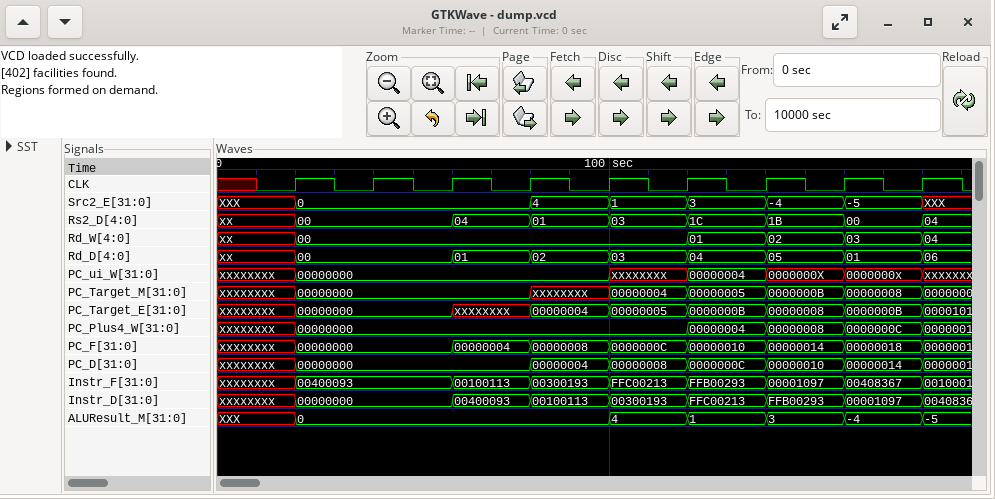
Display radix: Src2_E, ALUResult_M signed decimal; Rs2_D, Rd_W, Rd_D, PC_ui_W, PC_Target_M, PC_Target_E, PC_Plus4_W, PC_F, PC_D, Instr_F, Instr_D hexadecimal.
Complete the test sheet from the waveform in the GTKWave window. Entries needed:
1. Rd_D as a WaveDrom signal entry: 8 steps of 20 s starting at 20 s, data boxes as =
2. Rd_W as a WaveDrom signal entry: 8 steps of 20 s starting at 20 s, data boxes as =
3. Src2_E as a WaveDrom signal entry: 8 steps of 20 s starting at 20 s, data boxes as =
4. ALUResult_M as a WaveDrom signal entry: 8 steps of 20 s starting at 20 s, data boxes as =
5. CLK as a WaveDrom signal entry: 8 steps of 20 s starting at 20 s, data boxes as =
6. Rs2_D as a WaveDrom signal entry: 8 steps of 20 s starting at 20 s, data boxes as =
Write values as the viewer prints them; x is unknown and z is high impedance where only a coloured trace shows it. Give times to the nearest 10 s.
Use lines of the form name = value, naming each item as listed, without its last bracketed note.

Rd_D as a WaveDrom signal entry: 8 steps of 20 s starting at 20 s, data boxes as = = {name: 'Rd_D', wave: '=.======', data: '00 01 02 03 04 05 01'}
Rd_W as a WaveDrom signal entry: 8 steps of 20 s starting at 20 s, data boxes as = = {name: 'Rd_W', wave: '=....===', data: '00 01 02 03'}
Src2_E as a WaveDrom signal entry: 8 steps of 20 s starting at 20 s, data boxes as = = {name: 'Src2_E', wave: '=..=====', data: '0 4 1 3 -4 -5'}
ALUResult_M as a WaveDrom signal entry: 8 steps of 20 s starting at 20 s, data boxes as = = {name: 'ALUResult_M', wave: '=...====', data: '0 4 1 3 -4'}
CLK as a WaveDrom signal entry: 8 steps of 20 s starting at 20 s, data boxes as = = {name: 'CLK', wave: 'p.......'}
Rs2_D as a WaveDrom signal entry: 8 steps of 20 s starting at 20 s, data boxes as = = {name: 'Rs2_D', wave: '=.======', data: '00 04 01 03 1C 1B 00'}
